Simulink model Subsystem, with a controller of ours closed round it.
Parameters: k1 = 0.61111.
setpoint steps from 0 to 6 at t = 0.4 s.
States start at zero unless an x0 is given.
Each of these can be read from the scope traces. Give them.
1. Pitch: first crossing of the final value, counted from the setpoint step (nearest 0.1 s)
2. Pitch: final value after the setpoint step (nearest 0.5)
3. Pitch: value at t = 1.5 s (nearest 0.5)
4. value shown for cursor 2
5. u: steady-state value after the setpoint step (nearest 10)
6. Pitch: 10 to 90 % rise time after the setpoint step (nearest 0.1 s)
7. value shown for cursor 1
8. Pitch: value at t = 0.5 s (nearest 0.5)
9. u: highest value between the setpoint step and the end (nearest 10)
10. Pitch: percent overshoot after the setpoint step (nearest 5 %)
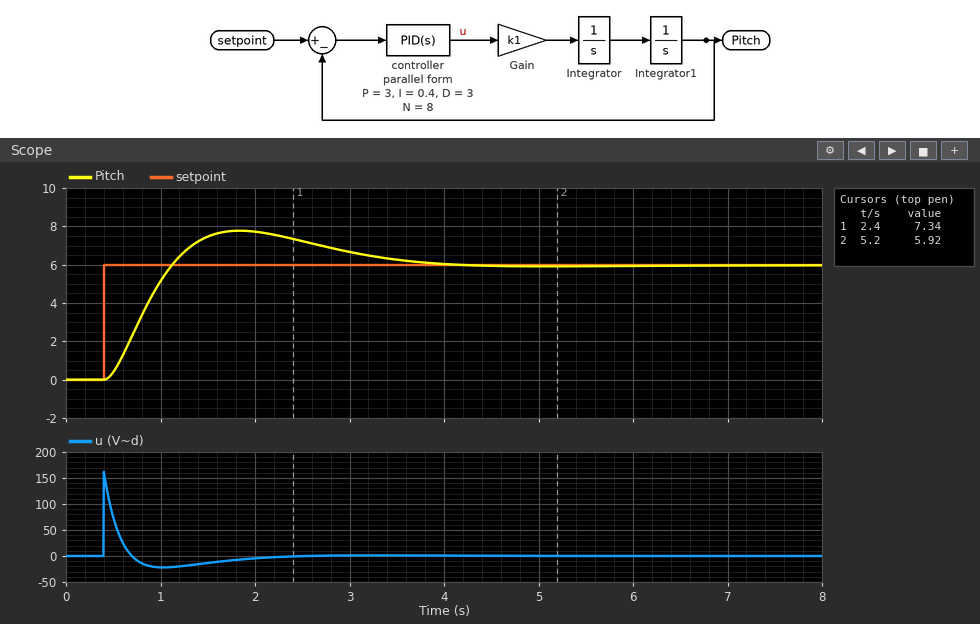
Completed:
0.7 s
6.0
7.5
5.92
0
0.5 s
7.34
0.5
160
30 %
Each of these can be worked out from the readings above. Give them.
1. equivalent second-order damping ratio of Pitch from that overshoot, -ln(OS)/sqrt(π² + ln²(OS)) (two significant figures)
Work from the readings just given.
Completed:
0.36
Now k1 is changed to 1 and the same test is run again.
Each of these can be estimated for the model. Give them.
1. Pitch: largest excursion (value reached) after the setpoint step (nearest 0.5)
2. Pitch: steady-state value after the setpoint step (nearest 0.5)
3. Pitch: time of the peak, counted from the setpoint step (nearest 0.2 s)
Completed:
7.5
6.0
1.0 s
